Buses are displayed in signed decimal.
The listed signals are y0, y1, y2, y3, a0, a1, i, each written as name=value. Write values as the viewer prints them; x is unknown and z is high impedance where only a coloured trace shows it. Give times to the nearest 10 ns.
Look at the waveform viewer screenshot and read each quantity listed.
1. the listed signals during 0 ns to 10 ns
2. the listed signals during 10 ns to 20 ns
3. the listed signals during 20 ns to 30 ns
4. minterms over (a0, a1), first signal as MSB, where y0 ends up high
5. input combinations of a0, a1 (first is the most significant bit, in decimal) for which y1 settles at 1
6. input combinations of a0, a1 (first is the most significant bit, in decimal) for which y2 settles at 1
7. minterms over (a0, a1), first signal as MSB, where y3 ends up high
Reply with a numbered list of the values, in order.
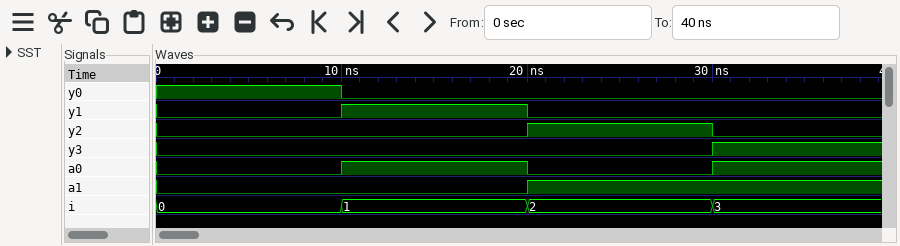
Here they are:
1. y0=1, y1=0, y2=0, y3=0, a0=0, a1=0, i=0
2. y0=0, y1=1, y2=0, y3=0, a0=1, a1=0, i=1
3. y0=0, y1=0, y2=1, y3=0, a0=0, a1=1, i=2
4. 0
5. 2
6. 1
7. 3
